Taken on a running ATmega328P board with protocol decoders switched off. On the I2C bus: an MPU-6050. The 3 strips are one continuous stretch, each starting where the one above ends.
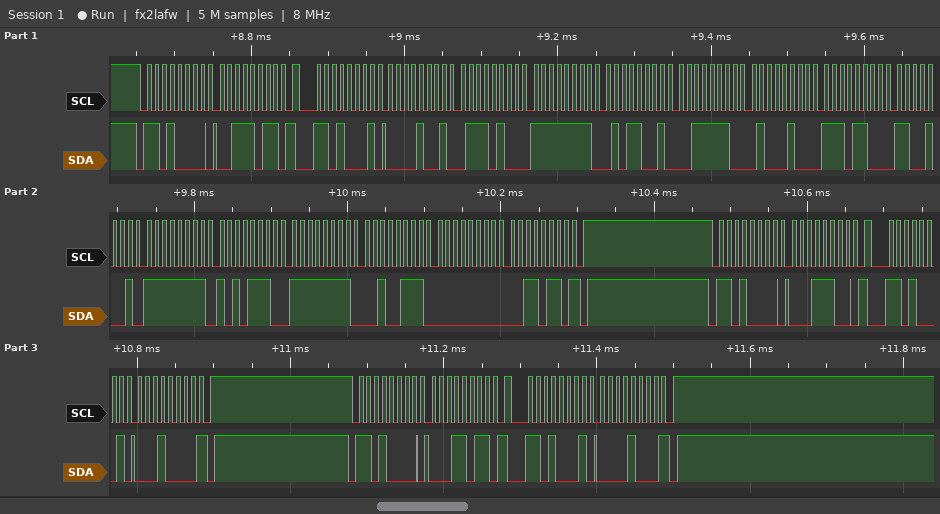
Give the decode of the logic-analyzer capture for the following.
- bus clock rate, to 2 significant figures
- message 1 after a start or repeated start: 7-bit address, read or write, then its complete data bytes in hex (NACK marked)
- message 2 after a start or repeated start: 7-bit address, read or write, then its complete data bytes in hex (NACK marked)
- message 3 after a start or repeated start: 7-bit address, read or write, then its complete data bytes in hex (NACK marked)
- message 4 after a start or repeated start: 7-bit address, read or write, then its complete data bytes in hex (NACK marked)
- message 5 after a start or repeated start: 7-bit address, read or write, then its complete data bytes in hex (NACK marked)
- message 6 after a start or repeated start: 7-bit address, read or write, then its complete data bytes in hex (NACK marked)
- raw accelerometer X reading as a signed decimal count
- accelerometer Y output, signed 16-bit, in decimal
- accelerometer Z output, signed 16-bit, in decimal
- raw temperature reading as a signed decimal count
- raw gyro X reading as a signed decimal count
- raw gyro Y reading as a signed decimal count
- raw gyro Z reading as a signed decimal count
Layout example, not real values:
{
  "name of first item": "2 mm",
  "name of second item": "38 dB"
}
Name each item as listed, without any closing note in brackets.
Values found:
{
  "bus clock rate, to 2 significant figures": "100 kHz",
  "message 1 after a start or repeated start: 7-bit address, read or write, then its complete data bytes in hex": "0x68 write: 3B",
  "message 2 after a start or repeated start: 7-bit address, read or write, then its complete data bytes in hex": "0x68 read: 09 74 FF 59 3E 44 EC C9 FF AE FF 27 00 36 NACK",
  "message 3 after a start or repeated start: 7-bit address, read or write, then its complete data bytes in hex": "0x68 write: 1C",
  "message 4 after a start or repeated start: 7-bit address, read or write, then its complete data bytes in hex": "0x68 read: 10 NACK",
  "message 5 after a start or repeated start: 7-bit address, read or write, then its complete data bytes in hex": "0x68 write: 1B",
  "message 6 after a start or repeated start: 7-bit address, read or write, then its complete data bytes in hex": "0x68 read: 08 NACK",
  "raw accelerometer X reading as a signed decimal count": "2420",
  "accelerometer Y output, signed 16-bit, in decimal": "-167",
  "accelerometer Z output, signed 16-bit, in decimal": "15940",
  "raw temperature reading as a signed decimal count": "-4919",
  "raw gyro X reading as a signed decimal count": "-82",
  "raw gyro Y reading as a signed decimal count": "-217",
  "raw gyro Z reading as a signed decimal count": "54"
}
